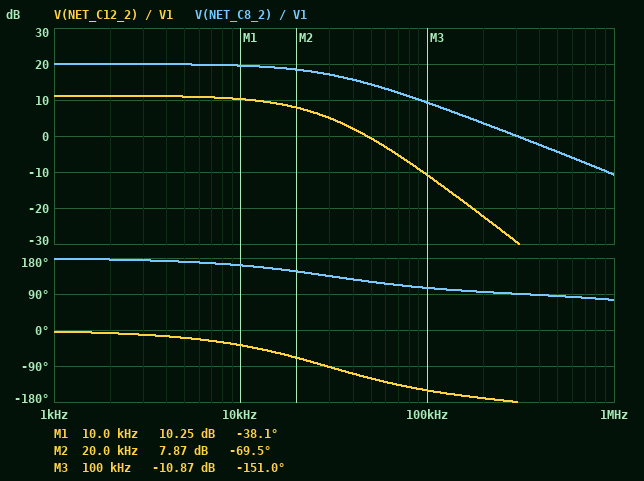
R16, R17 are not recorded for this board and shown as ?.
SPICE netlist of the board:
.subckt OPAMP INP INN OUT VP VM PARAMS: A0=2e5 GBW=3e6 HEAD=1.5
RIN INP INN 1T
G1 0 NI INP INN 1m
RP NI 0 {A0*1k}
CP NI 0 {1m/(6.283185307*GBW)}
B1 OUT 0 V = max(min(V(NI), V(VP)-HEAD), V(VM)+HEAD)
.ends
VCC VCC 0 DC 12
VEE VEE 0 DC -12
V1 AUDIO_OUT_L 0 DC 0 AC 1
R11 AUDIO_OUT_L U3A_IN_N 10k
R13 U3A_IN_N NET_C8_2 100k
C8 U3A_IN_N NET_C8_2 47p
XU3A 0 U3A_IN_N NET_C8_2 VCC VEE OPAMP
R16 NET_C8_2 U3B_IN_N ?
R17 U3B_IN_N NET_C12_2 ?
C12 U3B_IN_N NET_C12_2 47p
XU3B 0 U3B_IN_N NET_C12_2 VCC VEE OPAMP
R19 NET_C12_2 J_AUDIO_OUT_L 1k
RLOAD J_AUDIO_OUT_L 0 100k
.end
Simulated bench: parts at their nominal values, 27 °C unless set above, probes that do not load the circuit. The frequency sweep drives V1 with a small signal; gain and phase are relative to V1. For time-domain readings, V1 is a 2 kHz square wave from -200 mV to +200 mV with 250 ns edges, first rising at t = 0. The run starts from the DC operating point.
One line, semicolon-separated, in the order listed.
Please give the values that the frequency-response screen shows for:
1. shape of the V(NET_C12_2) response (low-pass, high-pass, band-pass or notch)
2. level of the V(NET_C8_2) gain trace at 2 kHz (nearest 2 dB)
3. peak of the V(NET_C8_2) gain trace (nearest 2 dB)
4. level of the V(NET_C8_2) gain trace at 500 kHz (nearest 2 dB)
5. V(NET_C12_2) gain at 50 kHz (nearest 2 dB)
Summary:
low-pass; 20 dB; 20 dB; -4 dB; 0 dB
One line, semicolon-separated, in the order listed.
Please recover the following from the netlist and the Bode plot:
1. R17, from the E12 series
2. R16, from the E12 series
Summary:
120 kΩ; 330 kΩ
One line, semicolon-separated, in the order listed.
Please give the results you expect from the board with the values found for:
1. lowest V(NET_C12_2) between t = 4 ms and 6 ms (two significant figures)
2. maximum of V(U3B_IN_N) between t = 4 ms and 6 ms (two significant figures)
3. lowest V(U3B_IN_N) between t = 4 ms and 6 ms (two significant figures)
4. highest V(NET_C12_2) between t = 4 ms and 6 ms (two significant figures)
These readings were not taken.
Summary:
-730 mV; 5.3 mV; -5.3 mV; 730 mV
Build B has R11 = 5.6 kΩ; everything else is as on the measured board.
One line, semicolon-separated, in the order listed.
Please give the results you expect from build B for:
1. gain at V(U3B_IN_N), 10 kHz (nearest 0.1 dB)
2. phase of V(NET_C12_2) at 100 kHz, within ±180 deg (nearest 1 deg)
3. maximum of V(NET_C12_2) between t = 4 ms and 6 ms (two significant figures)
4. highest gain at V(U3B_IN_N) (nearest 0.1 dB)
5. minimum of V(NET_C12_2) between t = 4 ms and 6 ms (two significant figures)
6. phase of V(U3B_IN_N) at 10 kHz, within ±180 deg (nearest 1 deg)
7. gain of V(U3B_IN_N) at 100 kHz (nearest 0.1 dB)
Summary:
-34.3 dB; -152 deg; 1.3 V; -30.3 dB; -1.3 V; -130 deg; -36.0 dB
